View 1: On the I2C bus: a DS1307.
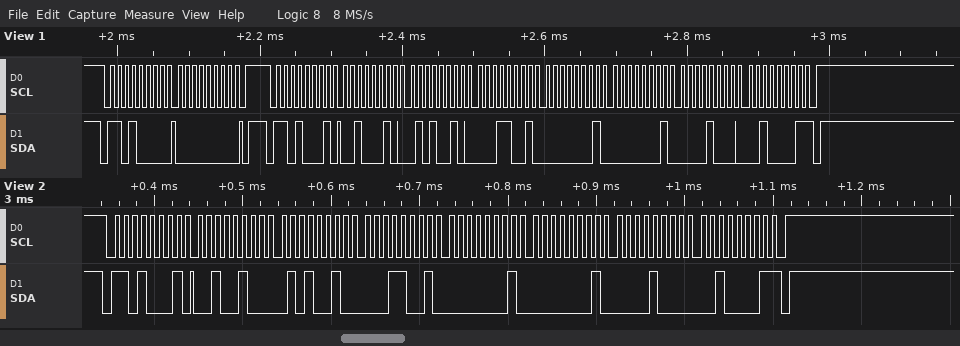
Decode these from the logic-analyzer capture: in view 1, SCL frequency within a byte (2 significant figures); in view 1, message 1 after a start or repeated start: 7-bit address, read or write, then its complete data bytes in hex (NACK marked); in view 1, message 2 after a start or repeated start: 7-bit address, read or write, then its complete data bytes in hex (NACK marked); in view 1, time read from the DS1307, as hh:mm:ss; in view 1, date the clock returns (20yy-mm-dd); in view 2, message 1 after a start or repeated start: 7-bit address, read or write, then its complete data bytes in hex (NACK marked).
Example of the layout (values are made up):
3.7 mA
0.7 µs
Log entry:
100 kHz
0x68 write: 00
0x68 read: 22 52 19 01 01 08 21 NACK
19:52:22
2021-08-01
0x68 read: 24 52 19 01 01 08 21 NACK
